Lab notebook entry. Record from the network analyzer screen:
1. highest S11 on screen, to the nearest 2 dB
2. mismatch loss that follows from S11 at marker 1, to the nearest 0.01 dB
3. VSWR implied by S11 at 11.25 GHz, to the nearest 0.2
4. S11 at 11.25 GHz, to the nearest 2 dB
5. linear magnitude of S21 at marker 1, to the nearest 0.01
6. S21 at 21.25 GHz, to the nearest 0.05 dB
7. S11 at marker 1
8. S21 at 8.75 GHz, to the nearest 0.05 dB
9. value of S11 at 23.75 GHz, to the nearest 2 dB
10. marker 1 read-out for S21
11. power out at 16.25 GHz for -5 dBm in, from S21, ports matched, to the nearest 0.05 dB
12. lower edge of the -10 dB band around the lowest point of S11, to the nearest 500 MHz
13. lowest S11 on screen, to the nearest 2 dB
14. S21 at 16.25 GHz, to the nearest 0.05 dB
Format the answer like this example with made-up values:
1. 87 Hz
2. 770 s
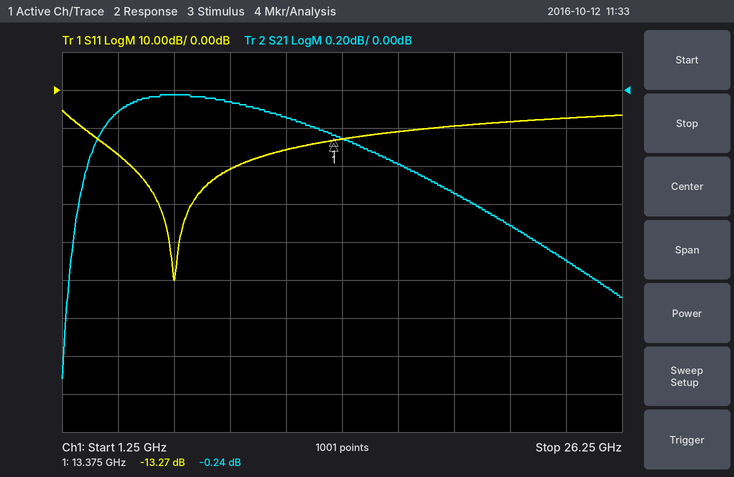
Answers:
1. -6 dB
2. 0.21 dB
3. 1.4
4. -16 dB
5. 0.97
6. -0.70 dB
7. -13.27 dB
8. -0.05 dB
9. -8 dB
10. -0.24 dB
11. -5.40 dBm
12. 2.0 GHz
13. -50 dB
14. -0.40 dB
